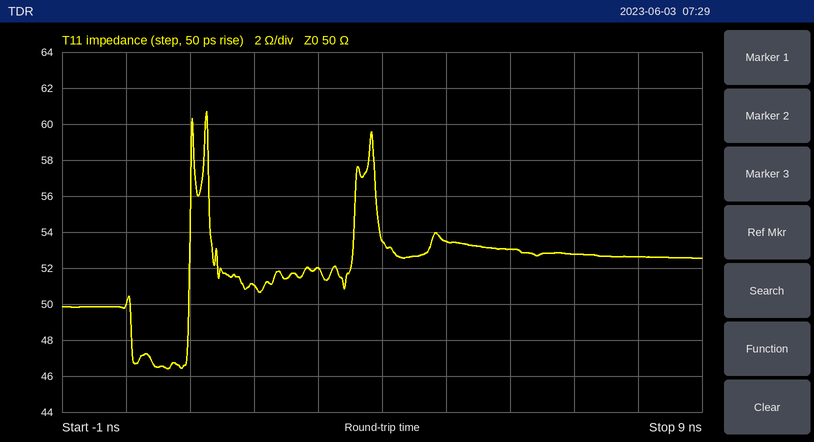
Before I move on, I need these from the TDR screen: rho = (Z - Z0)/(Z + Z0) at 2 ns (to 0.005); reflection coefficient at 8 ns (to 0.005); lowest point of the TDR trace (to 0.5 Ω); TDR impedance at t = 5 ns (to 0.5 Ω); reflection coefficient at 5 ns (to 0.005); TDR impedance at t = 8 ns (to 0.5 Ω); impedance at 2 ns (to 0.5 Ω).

+0.010
+0.025
46.5 Ω
53.5 Ω
+0.035
52.5 Ω
51.0 Ω
